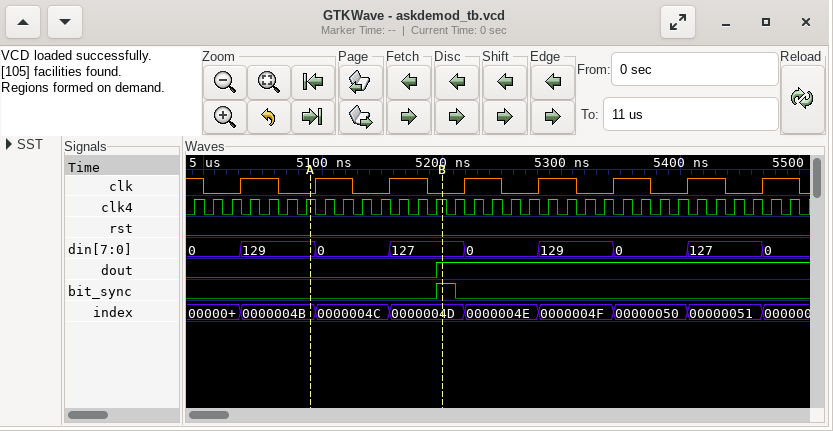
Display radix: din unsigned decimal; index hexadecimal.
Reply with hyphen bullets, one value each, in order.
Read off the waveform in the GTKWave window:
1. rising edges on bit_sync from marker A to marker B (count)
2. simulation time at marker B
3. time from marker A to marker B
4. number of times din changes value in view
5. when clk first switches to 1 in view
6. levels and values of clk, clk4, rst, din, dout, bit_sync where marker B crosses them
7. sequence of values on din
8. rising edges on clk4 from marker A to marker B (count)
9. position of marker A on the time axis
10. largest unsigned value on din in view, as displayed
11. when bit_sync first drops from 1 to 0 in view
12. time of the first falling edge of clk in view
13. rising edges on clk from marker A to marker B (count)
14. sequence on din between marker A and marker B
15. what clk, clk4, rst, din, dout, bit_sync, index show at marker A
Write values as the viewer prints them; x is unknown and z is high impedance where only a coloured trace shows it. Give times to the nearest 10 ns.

- 1
- 5200 ns
- 110 ns
- 8
- 5030 ns
- clk=0, clk4=1, rst=0, din=127, dout=1, bit_sync=1
- 0, 129, 0, 127, 0, 129, 0, 127, 0
- 7
- 5090 ns
- 129
- 5210 ns
- 5000 ns
- 2
- 129, 0, 127
- clk=0, clk4=1, rst=0, din=129, dout=0, bit_sync=0, index=0000004B
